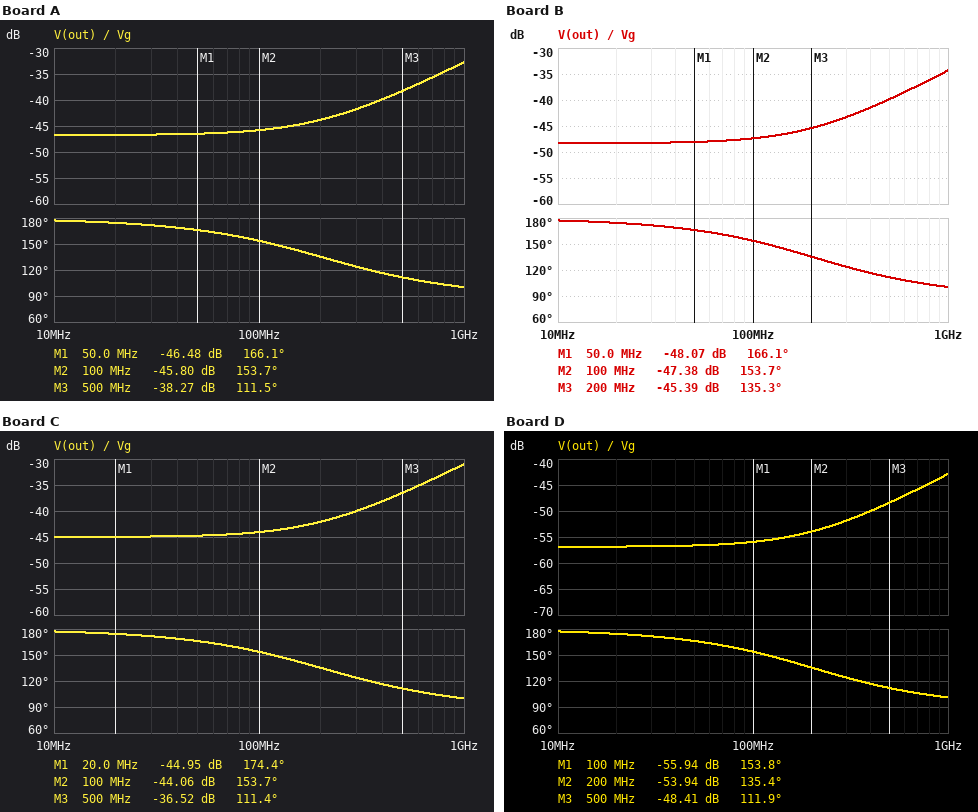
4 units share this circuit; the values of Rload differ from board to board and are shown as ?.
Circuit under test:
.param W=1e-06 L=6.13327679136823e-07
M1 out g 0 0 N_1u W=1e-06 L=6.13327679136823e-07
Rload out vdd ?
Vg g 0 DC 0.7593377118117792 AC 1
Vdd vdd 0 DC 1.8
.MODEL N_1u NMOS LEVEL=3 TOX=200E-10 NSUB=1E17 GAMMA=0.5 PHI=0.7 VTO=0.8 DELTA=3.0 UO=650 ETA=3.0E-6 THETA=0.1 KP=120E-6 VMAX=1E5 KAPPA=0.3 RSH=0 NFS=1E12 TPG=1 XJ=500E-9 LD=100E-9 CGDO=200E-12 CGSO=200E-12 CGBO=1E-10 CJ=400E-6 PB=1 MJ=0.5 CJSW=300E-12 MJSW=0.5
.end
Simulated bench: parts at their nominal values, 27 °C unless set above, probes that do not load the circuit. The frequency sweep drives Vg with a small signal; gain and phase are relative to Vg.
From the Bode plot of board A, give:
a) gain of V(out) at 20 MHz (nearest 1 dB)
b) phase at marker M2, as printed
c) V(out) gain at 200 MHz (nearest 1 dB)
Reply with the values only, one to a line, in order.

-47 dB
153.7 deg
-44 dB
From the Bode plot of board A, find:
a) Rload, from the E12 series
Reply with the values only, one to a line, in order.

18 kΩ
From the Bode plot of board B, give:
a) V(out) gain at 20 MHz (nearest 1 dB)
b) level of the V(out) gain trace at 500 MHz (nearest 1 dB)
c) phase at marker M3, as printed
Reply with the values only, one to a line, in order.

-48 dB
-40 dB
135.3 deg
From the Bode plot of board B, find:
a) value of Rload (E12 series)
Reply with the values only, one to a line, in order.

15 kΩ
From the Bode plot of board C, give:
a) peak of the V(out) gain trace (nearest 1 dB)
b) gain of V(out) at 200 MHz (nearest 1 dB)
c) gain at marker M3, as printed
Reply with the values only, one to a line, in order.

-31 dB
-42 dB
-36.52 dB
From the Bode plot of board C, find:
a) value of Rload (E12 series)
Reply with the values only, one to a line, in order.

22 kΩ
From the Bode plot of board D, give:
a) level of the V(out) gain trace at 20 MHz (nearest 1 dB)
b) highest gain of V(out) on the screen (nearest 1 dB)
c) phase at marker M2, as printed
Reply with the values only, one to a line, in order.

-57 dB
-43 dB
135.4 deg
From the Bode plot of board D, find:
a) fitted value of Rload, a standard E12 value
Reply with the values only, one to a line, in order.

5.6 kΩ
